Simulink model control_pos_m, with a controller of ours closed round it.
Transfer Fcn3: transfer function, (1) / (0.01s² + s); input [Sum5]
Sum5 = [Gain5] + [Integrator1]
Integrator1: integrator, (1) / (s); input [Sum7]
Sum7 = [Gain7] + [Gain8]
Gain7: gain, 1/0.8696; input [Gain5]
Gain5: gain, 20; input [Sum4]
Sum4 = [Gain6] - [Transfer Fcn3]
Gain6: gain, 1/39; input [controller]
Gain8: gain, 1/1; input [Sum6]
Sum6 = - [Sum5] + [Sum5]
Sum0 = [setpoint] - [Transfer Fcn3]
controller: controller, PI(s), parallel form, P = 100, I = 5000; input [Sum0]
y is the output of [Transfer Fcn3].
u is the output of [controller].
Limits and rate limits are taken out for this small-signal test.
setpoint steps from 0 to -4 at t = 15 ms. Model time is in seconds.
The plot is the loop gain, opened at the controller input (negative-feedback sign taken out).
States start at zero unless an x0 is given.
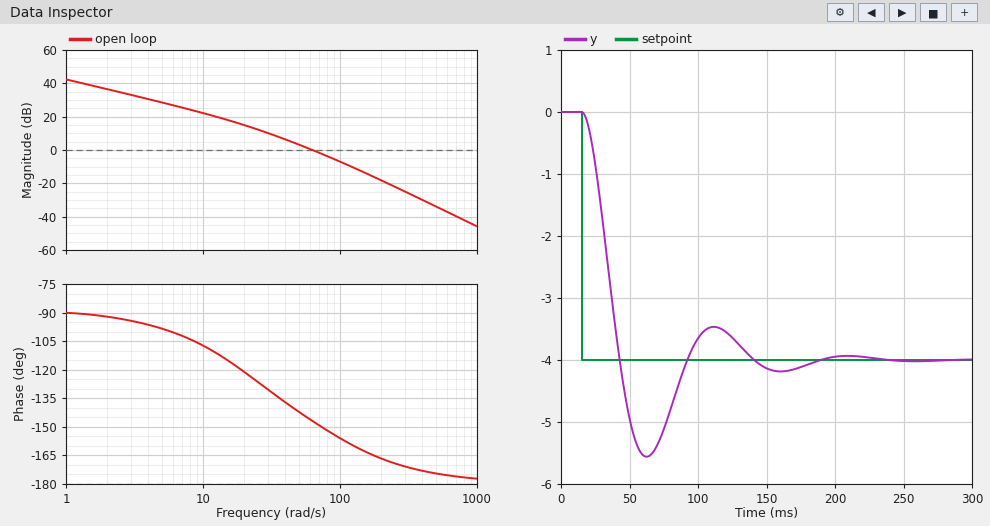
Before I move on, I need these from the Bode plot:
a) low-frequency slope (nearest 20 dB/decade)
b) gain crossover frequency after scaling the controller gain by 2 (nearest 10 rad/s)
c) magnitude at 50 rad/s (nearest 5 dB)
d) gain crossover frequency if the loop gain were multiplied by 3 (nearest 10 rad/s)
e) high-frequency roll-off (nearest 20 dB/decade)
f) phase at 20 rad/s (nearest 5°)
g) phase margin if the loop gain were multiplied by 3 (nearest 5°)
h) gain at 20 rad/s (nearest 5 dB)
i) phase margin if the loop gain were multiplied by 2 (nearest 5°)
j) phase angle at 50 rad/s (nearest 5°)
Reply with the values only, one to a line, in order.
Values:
-20 dB/decade
90 rad/s
5 dB
120 rad/s
-40 dB/decade
-120°
20°
15 dB
25°
-140°
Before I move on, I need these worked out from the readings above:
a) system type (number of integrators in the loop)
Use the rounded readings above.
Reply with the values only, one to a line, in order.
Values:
1
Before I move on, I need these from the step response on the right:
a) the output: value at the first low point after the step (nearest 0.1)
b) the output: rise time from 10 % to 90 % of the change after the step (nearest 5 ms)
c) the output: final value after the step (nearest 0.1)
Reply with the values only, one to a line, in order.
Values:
-5.6
20 ms
-4.0
